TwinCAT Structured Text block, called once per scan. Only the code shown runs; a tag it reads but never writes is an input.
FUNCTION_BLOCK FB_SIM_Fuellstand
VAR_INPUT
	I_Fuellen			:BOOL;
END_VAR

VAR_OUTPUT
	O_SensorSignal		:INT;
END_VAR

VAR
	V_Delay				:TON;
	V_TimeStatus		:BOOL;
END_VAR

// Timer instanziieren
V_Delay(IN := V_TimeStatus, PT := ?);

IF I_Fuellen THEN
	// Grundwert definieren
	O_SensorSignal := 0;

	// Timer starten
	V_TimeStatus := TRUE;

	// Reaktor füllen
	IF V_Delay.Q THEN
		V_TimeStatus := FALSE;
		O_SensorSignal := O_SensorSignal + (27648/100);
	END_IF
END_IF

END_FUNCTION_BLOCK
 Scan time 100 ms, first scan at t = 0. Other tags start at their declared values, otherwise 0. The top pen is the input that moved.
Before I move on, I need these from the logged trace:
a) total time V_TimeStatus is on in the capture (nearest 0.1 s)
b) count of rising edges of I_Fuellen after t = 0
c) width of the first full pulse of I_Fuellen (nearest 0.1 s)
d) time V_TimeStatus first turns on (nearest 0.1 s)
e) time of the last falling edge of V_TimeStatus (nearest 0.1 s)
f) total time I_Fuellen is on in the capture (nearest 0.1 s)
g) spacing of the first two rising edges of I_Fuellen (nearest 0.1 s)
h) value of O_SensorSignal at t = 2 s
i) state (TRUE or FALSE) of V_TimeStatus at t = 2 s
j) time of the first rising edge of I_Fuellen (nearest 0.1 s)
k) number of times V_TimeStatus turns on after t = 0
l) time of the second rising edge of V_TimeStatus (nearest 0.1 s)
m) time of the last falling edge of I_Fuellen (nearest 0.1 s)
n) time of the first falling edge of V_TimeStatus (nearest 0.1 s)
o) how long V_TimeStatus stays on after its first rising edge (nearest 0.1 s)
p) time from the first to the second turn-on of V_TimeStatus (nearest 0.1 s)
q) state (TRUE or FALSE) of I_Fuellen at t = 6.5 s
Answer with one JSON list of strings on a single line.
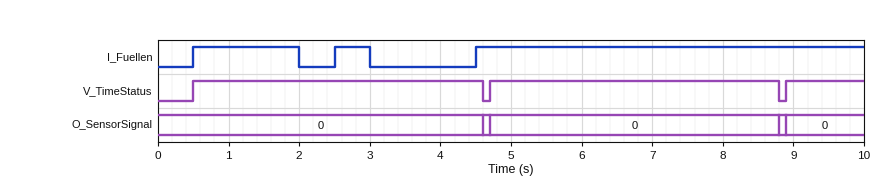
["9.3 s", "3", "1.5 s", "0.5 s", "8.8 s", "7.5 s", "2.0 s", "0", "TRUE", "0.5 s", "3", "4.7 s", "3.0 s", "4.6 s", "4.1 s", "4.2 s", "TRUE"]
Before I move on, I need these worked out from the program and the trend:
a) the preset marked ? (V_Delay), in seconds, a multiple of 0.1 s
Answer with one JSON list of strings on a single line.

["4.0 s"]
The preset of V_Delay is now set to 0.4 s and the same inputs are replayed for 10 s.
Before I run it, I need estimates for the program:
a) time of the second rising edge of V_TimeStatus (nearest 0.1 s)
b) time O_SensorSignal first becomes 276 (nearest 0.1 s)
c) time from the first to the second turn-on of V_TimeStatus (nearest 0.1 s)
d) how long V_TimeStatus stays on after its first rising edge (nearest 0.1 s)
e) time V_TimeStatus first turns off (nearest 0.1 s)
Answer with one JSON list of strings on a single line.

["1.1 s", "1.0 s", "0.6 s", "0.5 s", "1.0 s"]
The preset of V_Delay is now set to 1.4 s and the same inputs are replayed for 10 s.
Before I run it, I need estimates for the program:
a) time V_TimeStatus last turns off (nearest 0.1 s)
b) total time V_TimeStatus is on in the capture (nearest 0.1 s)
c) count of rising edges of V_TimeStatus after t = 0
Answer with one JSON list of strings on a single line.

["9.3 s", "9.0 s", "6"]
